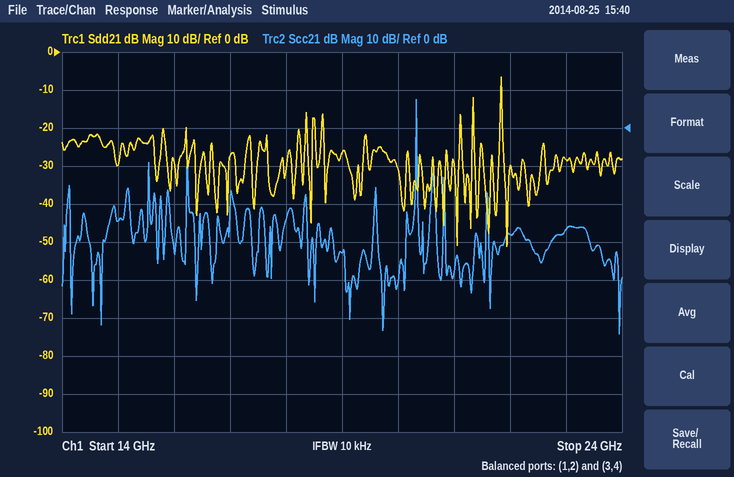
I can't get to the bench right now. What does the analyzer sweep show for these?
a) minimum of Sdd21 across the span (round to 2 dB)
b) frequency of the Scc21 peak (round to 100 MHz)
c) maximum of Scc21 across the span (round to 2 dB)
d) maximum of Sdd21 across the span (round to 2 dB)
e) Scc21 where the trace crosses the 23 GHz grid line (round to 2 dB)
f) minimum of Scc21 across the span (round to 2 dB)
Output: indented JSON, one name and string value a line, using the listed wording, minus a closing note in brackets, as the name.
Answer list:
{
  "minimum of Sdd21 across the span": "-52 dB",
  "frequency of the Scc21 peak": "20.3 GHz",
  "maximum of Scc21 across the span": "8 dB",
  "maximum of Sdd21 across the span": "-6 dB",
  "Scc21 where the trace crosses the 23 GHz grid line": "-26 dB",
  "minimum of Scc21 across the span": "-54 dB"
}
